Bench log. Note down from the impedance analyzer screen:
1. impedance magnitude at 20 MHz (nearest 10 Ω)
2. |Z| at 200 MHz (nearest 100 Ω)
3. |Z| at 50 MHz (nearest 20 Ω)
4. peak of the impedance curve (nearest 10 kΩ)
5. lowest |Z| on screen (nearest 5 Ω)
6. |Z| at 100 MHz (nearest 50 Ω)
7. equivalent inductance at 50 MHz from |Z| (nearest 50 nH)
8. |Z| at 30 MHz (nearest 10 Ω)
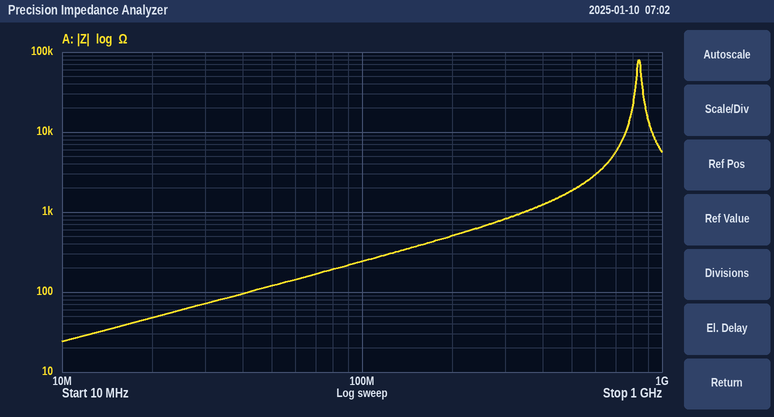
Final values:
50 Ω
500 Ω
120 Ω
80 kΩ
25 Ω
250 Ω
400 nH
70 Ω
